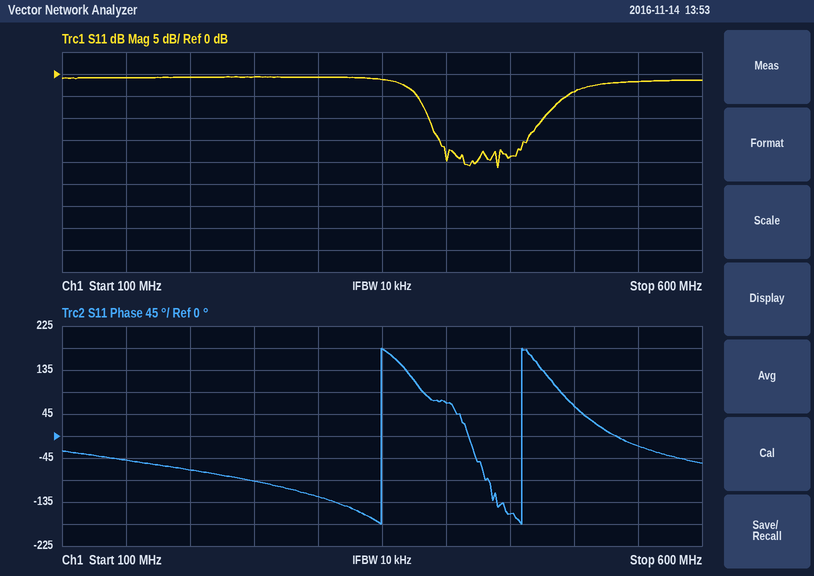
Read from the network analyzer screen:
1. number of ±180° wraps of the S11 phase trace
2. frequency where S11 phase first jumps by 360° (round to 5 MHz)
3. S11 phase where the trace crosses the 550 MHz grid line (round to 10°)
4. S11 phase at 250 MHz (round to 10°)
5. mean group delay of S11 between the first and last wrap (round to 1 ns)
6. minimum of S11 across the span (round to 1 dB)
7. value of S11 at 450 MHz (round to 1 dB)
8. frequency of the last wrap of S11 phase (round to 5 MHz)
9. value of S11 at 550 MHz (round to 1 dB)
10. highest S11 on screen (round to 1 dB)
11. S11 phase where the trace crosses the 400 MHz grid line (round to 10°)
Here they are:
2
350 MHz
-20°
-90°
9 ns
-21 dB
-19 dB
460 MHz
-2 dB
-1 dB
70°
